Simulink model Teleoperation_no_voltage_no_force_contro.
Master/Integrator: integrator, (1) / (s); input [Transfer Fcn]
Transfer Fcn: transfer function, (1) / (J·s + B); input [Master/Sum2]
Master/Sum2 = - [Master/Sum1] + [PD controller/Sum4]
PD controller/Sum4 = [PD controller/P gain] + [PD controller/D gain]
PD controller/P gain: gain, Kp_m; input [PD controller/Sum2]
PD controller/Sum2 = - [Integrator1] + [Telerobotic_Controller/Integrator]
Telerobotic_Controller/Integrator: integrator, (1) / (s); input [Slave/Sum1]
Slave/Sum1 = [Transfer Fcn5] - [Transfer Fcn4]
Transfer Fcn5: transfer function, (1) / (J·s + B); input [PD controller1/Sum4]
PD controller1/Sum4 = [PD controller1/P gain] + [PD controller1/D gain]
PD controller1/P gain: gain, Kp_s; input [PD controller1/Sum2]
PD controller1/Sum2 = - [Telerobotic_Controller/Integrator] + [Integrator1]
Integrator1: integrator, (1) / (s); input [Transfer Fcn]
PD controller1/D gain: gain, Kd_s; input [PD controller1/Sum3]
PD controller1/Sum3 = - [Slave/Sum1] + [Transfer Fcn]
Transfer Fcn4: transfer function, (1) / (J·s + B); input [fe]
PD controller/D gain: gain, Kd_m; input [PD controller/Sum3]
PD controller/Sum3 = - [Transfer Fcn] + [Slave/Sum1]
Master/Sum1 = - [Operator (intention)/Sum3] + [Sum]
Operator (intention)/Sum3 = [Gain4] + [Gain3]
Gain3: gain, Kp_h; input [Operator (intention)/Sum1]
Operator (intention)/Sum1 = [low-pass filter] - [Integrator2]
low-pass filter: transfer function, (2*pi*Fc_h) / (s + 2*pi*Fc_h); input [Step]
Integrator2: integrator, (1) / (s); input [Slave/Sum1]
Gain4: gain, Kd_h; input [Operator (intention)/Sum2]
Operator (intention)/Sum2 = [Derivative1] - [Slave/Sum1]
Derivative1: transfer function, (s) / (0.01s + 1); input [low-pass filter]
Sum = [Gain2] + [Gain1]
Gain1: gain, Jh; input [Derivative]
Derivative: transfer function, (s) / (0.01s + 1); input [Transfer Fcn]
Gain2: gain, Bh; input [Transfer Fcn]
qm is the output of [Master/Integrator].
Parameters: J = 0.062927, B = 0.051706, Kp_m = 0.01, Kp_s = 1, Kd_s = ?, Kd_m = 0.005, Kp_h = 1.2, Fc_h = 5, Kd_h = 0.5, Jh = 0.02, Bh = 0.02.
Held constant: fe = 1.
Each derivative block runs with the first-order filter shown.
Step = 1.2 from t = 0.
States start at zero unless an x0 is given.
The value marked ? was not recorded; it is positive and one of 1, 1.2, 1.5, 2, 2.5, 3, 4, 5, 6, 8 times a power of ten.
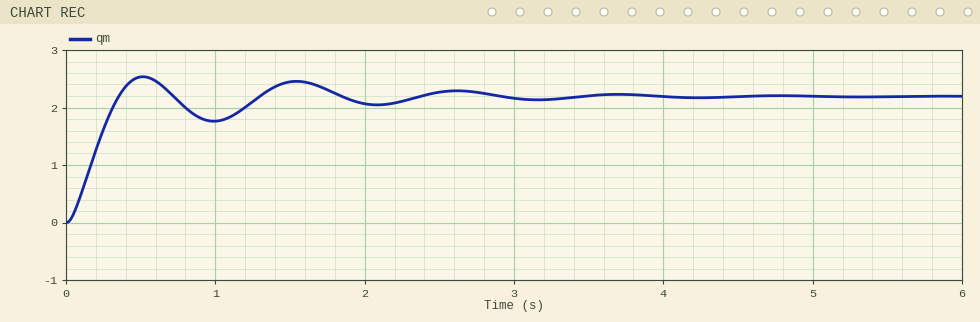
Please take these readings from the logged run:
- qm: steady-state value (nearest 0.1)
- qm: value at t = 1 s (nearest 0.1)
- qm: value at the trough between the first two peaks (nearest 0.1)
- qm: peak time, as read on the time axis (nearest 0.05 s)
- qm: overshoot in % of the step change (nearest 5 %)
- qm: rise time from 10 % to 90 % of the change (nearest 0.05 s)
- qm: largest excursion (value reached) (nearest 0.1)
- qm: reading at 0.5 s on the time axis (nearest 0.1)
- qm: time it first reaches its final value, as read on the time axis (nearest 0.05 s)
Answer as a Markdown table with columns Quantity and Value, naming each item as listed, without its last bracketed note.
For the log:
| Quantity | Value |
|---|---|
| qm: steady-state value | 2.2 |
| qm: value at t = 1 s | 1.8 |
| qm: value at the trough between the first two peaks | 1.8 |
| qm: peak time, as read on the time axis | 0.50 s |
| qm: overshoot in % of the step change | 15 % |
| qm: rise time from 10 % to 90 % of the change | 0.25 s |
| qm: largest excursion (value reached) | 2.5 |
| qm: reading at 0.5 s on the time axis | 2.5 |
| qm: time it first reaches its final value, as read on the time axis | 0.35 s |
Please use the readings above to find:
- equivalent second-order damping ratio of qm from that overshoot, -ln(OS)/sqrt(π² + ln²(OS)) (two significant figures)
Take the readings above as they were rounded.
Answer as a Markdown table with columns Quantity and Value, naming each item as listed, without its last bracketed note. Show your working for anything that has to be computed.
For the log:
| Quantity | Value |
|---|---|
| equivalent second-order damping ratio of qm from that overshoot, -ln(OS)/sqrt(π² + ln²(OS)) | ln(0.15) = -1.897; 1.897 / sqrt(9.870 + 3.599) = 0.52 |
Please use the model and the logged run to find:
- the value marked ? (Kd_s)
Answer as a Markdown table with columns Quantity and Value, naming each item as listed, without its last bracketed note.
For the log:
| Quantity | Value |
|---|---|
| the value marked ? | 0.3 |
